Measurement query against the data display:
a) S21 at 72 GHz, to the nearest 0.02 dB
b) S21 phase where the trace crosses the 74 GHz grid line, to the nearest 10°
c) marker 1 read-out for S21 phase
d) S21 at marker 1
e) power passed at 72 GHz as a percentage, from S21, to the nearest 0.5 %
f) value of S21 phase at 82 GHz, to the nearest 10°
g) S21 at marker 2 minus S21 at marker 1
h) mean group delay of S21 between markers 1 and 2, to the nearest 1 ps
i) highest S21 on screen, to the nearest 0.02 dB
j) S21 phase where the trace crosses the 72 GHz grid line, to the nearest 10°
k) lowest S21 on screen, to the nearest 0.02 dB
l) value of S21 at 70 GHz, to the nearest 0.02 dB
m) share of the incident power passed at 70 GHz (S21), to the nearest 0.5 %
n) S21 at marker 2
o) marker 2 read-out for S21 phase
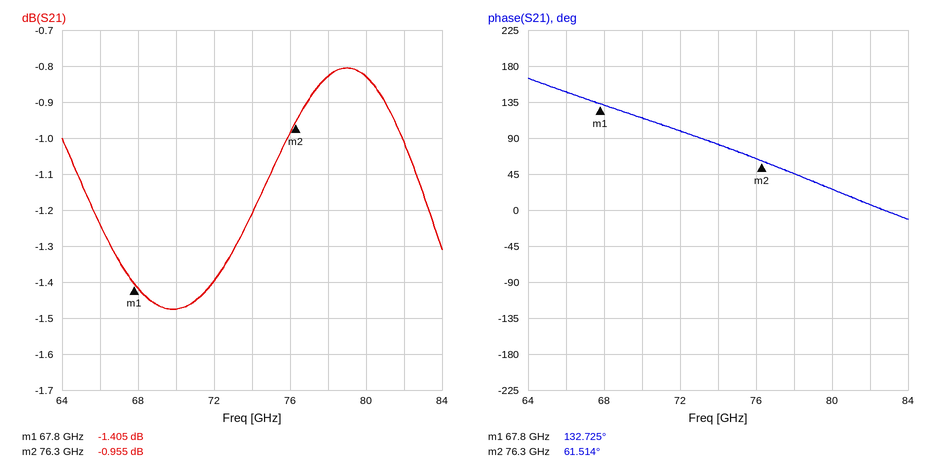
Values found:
-1.40 dB
80°
132.725°
-1.405 dB
72.5 %
10°
0.450 dB
23 ps
-0.80 dB
100°
-1.48 dB
-1.48 dB
71.0 %
-0.955 dB
61.514°
